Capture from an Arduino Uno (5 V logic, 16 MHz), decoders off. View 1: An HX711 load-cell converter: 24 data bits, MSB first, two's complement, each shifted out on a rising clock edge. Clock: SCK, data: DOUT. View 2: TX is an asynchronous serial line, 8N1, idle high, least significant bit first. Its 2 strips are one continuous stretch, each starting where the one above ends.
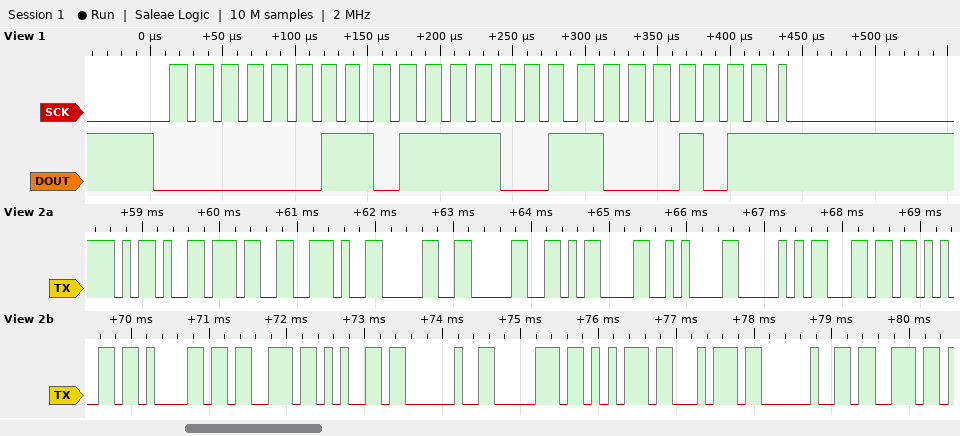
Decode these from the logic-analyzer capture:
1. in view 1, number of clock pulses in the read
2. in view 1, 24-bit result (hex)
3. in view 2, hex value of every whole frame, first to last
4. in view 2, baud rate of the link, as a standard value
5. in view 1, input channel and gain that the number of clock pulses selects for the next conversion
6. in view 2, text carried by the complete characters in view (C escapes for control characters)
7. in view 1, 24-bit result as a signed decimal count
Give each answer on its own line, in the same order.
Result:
25
0x03798B
2D 37 2E 30 30 0D 0A 50 6C 65 61 73 65 20 70 75 74 20 73
9600 baud
channel A, gain 128
"-7.00\r\nPlease put s"
227723
